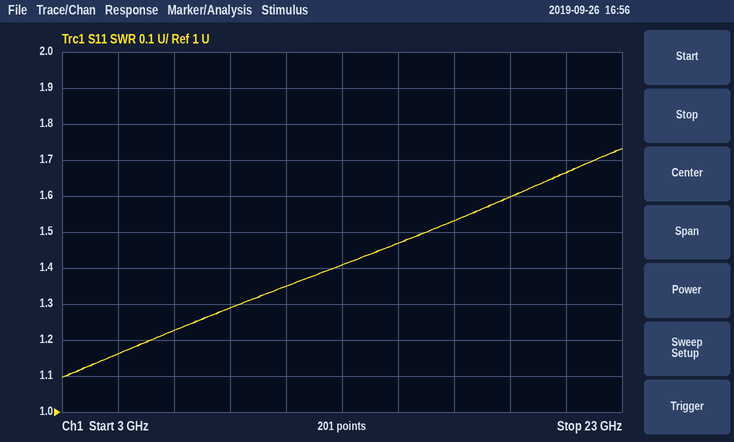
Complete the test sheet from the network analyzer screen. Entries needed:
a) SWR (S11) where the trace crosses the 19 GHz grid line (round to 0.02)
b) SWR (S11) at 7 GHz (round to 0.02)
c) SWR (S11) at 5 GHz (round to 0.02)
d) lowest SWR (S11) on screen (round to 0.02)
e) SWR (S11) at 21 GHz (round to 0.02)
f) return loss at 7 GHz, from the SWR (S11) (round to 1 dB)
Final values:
1.60
1.22
1.16
1.10
1.66
20 dB
